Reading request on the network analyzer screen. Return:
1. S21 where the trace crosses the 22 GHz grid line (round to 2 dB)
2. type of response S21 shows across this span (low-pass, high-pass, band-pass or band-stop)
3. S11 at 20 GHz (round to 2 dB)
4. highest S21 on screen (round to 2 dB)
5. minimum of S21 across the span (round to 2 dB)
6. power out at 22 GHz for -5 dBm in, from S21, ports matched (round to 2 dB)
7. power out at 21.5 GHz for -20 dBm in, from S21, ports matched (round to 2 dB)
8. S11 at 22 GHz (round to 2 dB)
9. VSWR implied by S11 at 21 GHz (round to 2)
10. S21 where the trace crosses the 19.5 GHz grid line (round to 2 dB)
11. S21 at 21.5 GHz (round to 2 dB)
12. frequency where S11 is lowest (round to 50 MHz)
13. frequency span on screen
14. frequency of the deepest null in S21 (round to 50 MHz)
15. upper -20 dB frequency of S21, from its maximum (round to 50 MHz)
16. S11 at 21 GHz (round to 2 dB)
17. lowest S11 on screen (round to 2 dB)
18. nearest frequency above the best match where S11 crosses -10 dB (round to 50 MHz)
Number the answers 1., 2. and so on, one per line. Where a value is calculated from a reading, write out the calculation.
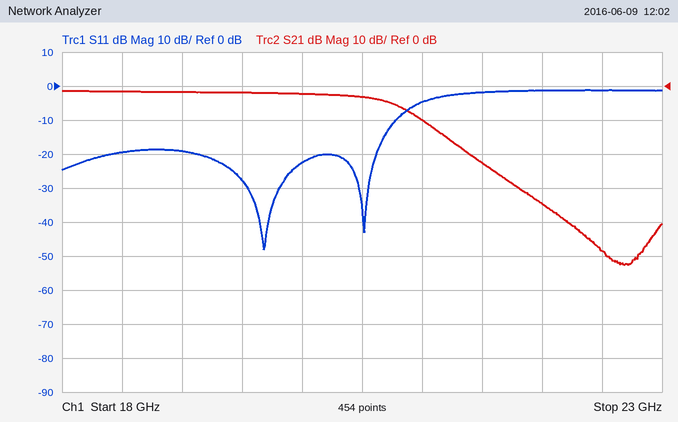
1. -34 dB
2. low-pass
3. -22 dB
4. -2 dB
5. -52 dB
6. -5 dBm + (-34 dB) = -40 dBm
7. -20 dBm + (-22 dB) = -42 dBm
8. -2 dB
9. |Γ| = 10^(-4/20) = 0.6310; VSWR = (1 + 0.6310)/(1 − 0.6310) ≈ 4
10. -2 dB
11. -22 dB
12. 19.70 GHz
13. 5 GHz
14. 22.70 GHz
15. 21.45 GHz
16. -4 dB
17. -48 dB
18. 20.80 GHz
